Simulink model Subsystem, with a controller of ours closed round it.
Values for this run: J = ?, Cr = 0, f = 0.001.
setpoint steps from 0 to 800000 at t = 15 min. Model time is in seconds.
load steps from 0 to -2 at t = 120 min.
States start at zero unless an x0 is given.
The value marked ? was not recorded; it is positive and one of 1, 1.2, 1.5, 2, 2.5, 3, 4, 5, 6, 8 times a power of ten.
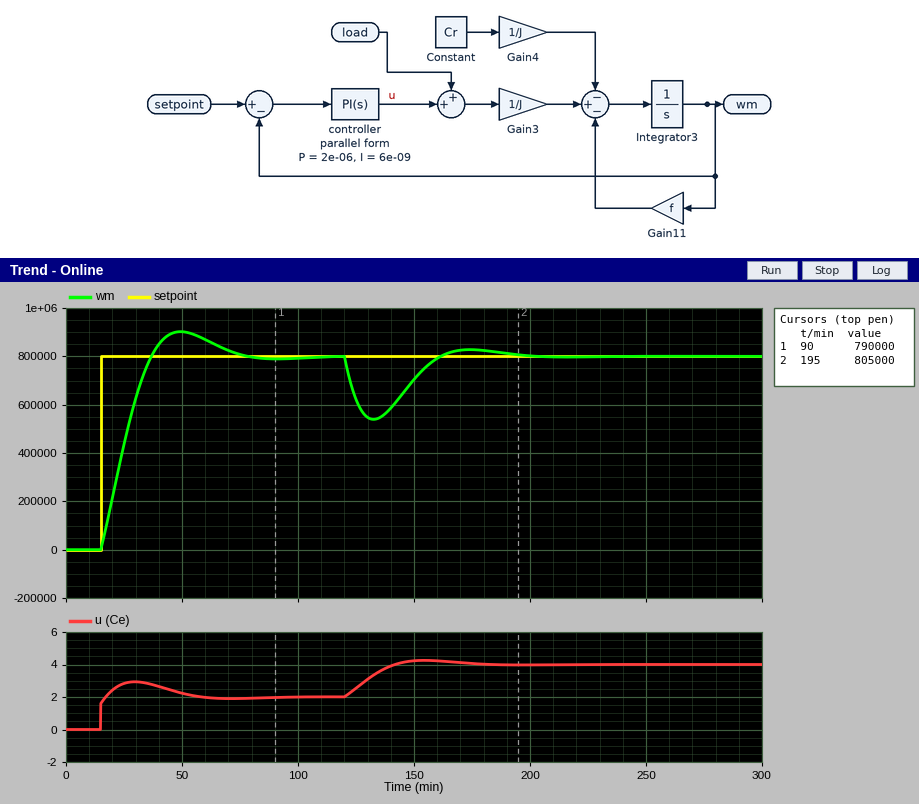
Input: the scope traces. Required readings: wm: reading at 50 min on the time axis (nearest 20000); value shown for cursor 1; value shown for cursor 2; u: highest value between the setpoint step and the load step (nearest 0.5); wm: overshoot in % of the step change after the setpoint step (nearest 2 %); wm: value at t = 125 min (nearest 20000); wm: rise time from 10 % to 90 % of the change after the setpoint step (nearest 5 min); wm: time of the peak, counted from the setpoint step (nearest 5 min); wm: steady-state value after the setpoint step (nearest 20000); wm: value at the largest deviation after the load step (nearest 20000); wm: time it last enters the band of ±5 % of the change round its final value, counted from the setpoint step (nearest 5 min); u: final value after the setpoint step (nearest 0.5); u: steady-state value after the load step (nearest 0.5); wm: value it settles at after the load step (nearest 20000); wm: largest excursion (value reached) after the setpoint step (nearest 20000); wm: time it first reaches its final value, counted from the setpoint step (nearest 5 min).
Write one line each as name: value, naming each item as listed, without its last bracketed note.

wm: reading at 50 min on the time axis: 900000
value shown for cursor 1: 790000
value shown for cursor 2: 805000
u: highest value between the setpoint step and the load step: 3.0
wm: overshoot in % of the step change after the setpoint step: 12 %
wm: value at t = 125 min: 620000
wm: rise time from 10 % to 90 % of the change after the setpoint step: 15 min
wm: time of the peak, counted from the setpoint step: 35 min
wm: steady-state value after the setpoint step: 800000
wm: value at the largest deviation after the load step: 540000
wm: time it last enters the band of ±5 % of the change round its final value, counted from the setpoint step: 50 min
u: final value after the setpoint step: 2.0
u: steady-state value after the load step: 4.0
wm: value it settles at after the load step: 800000
wm: largest excursion (value reached) after the setpoint step: 900000
wm: time it first reaches its final value, counted from the setpoint step: 20 min
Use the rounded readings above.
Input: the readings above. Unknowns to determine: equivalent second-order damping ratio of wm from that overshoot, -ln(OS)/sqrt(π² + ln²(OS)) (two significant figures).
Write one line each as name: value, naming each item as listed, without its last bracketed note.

equivalent second-order damping ratio of wm from that overshoot, -ln(OS)/sqrt(π² + ln²(OS)): 0.56
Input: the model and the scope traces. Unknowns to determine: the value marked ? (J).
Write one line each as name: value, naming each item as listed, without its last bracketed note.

the value marked ?: 0.0025
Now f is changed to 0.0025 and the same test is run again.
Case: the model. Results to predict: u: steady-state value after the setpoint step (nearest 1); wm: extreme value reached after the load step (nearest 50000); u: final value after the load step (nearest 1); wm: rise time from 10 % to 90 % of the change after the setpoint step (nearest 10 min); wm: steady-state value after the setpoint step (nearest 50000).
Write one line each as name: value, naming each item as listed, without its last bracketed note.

u: steady-state value after the setpoint step: 5
wm: extreme value reached after the load step: 600000
u: final value after the load step: 7
wm: rise time from 10 % to 90 % of the change after the setpoint step: 40 min
wm: steady-state value after the setpoint step: 800000
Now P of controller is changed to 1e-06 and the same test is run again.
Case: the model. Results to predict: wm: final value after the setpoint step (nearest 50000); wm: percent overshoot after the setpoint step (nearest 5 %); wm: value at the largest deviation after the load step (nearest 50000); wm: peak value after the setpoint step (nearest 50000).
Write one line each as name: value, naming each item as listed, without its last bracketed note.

wm: final value after the setpoint step: 800000
wm: percent overshoot after the setpoint step: 20 %
wm: value at the largest deviation after the load step: 500000
wm: peak value after the setpoint step: 950000
